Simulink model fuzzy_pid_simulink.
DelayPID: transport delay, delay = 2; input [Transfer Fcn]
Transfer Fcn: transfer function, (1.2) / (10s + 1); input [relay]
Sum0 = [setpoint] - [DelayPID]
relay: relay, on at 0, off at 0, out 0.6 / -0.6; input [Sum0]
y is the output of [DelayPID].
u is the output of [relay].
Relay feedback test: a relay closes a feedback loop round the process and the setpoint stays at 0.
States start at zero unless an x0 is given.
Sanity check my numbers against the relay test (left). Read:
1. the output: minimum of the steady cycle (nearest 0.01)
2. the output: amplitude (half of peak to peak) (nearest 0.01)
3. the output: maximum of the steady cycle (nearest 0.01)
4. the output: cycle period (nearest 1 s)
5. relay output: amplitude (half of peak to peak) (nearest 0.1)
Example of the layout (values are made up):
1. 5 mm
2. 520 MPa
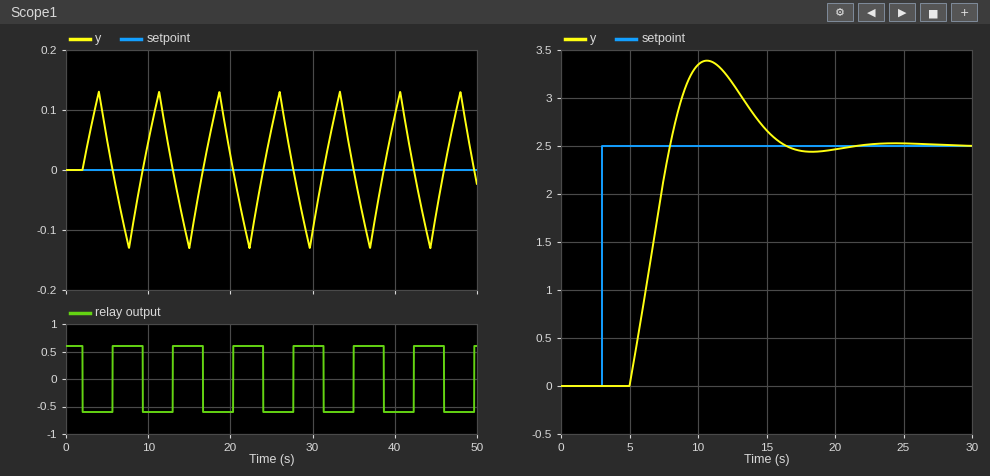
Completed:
1. -0.13
2. 0.13
3. 0.13
4. 7 s
5. 0.6
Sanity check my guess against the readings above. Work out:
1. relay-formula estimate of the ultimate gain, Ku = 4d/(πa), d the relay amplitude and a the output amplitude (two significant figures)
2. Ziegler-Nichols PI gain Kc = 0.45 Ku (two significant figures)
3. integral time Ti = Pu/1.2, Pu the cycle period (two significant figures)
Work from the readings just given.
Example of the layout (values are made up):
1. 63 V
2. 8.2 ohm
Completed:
1. 5.9
2. 2.7
3. 5.8 s
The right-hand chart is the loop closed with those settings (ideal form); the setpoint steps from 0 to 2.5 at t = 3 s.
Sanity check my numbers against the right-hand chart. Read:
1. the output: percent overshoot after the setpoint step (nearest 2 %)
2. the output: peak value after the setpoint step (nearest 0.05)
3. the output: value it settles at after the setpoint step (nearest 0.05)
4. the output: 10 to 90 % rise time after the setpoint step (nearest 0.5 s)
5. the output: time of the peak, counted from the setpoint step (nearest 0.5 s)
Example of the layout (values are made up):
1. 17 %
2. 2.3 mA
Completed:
1. 36 %
2. 3.40
3. 2.50
4. 2.5 s
5. 7.5 s
